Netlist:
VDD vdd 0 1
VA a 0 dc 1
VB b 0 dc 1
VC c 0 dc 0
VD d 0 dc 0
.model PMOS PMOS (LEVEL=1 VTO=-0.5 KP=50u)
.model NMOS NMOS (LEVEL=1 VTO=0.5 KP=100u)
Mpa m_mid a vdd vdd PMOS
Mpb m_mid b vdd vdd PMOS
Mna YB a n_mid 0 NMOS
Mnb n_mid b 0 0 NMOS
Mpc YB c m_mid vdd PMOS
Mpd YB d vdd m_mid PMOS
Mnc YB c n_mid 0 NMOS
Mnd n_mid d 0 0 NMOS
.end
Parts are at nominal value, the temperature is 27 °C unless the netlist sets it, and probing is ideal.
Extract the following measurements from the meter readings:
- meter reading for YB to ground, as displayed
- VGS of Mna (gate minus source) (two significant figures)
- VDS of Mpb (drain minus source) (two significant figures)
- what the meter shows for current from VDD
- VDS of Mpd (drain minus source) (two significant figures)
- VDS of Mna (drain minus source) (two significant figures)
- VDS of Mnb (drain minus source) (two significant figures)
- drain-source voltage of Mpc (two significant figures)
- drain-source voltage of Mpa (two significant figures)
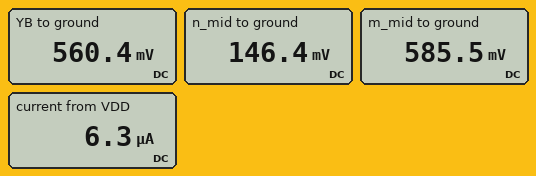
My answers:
560.4 mV
850 mV
-410 mV
6.3 µA
-440 mV
410 mV
150 mV
-25 mV
-410 mV
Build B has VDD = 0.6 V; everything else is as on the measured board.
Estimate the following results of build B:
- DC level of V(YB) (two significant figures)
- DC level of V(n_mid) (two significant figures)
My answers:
10 mV
5.0 mV
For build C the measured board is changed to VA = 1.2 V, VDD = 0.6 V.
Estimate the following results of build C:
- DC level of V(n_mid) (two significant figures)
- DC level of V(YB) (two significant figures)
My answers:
5.0 mV
8.6 mV
